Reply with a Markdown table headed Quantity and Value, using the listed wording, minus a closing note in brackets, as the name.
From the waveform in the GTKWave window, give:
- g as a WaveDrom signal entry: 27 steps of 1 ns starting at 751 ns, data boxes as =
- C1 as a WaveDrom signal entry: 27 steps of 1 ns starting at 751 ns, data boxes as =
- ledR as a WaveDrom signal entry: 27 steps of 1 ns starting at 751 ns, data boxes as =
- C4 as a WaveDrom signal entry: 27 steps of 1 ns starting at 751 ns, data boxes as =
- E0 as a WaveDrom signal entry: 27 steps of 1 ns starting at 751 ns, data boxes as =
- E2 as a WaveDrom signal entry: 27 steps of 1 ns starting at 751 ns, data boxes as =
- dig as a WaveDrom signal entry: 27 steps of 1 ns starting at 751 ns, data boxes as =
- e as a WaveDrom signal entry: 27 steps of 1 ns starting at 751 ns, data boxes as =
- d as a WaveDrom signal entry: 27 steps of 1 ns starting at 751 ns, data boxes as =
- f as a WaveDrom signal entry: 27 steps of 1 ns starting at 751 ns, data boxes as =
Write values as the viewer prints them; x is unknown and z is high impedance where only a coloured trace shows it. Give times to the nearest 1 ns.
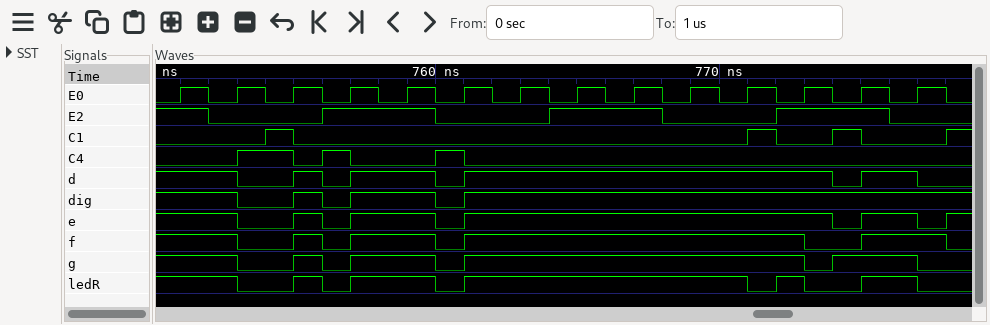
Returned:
| Quantity | Value |
|---|---|
| g as a WaveDrom signal entry: 27 steps of 1 ns starting at 751 ns, data boxes as = | {name: 'g', wave: '1.0.101..01...........01..0'} |
| C1 as a WaveDrom signal entry: 27 steps of 1 ns starting at 751 ns, data boxes as = | {name: 'C1', wave: '0..10...............10.10..'} |
| ledR as a WaveDrom signal entry: 27 steps of 1 ns starting at 751 ns, data boxes as = | {name: 'ledR', wave: '1.0.101..01.........010.1.0'} |
| C4 as a WaveDrom signal entry: 27 steps of 1 ns starting at 751 ns, data boxes as = | {name: 'C4', wave: '0.1.010..10................'} |
| E0 as a WaveDrom signal entry: 27 steps of 1 ns starting at 751 ns, data boxes as = | {name: 'E0', wave: '101010101010101010101010101'} |
| E2 as a WaveDrom signal entry: 27 steps of 1 ns starting at 751 ns, data boxes as = | {name: 'E2', wave: '10...1...0...1...0...1...0.'} |
| dig as a WaveDrom signal entry: 27 steps of 1 ns starting at 751 ns, data boxes as = | {name: 'dig', wave: '1.0.101..01................'} |
| e as a WaveDrom signal entry: 27 steps of 1 ns starting at 751 ns, data boxes as = | {name: 'e', wave: '1.0.101..01............01.0'} |
| d as a WaveDrom signal entry: 27 steps of 1 ns starting at 751 ns, data boxes as = | {name: 'd', wave: '1.0.101..01............01.0'} |
| f as a WaveDrom signal entry: 27 steps of 1 ns starting at 751 ns, data boxes as = | {name: 'f', wave: '1.0.101..01...........0.1..'} |
